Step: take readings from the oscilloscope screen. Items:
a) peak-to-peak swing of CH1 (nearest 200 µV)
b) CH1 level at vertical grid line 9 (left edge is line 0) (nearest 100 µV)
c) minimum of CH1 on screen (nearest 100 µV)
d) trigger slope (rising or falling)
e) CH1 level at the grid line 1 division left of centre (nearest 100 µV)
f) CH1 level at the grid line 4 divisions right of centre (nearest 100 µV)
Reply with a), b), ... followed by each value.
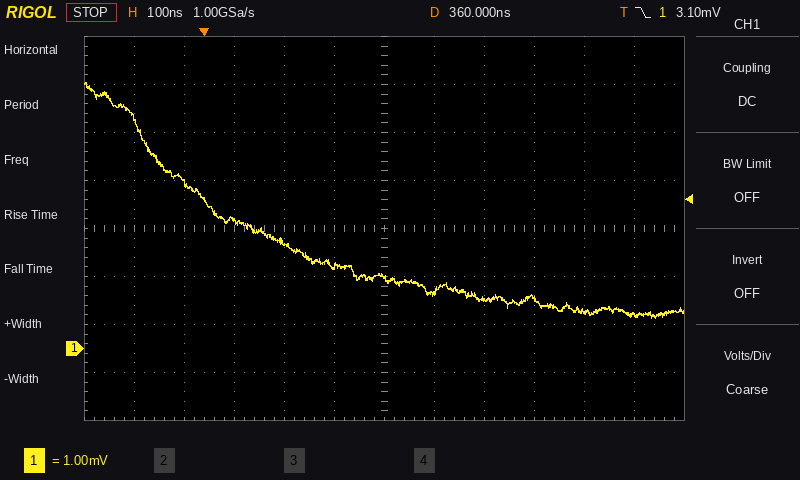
a) 5.0 mV
b) 1.0 mV
c) 600 µV
d) falling
e) 1.7 mV
f) 800 µV
